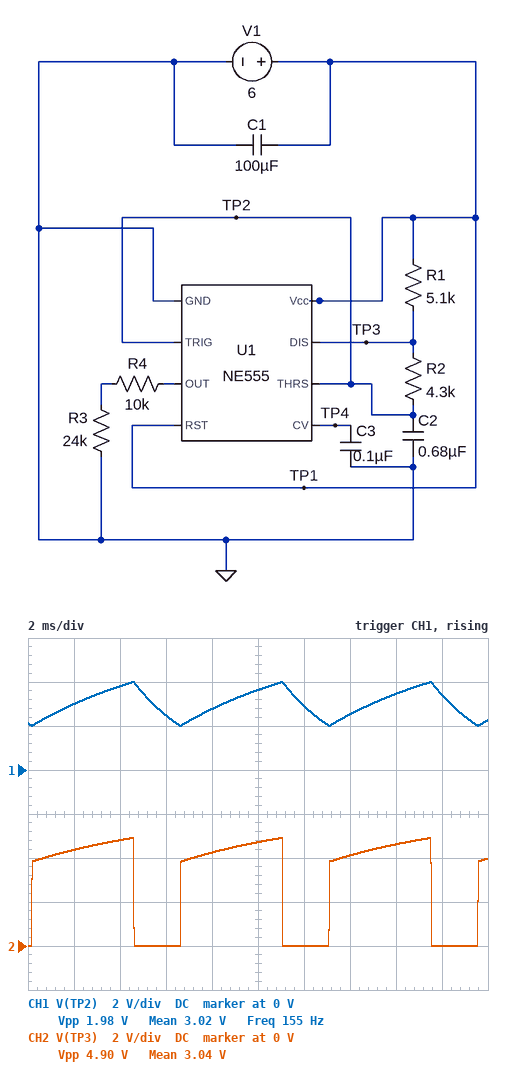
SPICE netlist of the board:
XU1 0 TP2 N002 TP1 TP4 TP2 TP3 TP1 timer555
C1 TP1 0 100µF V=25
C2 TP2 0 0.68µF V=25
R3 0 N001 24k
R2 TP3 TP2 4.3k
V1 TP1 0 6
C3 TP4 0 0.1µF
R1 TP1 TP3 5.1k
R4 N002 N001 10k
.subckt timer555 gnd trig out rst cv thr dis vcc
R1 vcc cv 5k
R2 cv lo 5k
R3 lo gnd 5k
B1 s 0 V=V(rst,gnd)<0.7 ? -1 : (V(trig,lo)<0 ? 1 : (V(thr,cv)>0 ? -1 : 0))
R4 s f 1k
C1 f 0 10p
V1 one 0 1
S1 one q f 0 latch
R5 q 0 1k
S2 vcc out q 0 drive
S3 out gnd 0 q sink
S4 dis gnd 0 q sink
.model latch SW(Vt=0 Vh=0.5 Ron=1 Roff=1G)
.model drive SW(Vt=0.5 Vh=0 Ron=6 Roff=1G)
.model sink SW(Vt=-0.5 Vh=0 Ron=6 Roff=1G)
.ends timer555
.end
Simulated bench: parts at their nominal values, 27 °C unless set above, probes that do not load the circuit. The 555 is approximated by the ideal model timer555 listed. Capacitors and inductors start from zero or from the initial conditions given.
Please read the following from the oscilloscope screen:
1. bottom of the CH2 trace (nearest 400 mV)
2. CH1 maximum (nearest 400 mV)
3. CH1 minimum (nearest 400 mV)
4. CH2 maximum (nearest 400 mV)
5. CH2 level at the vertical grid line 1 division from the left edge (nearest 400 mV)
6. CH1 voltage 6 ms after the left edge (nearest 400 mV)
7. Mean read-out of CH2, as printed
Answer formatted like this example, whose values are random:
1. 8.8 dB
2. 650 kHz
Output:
1. 0 V
2. 4.0 V
3. 2.0 V
4. 4.8 V
5. 4.4 V
6. 2.4 V
7. 3.04 V
